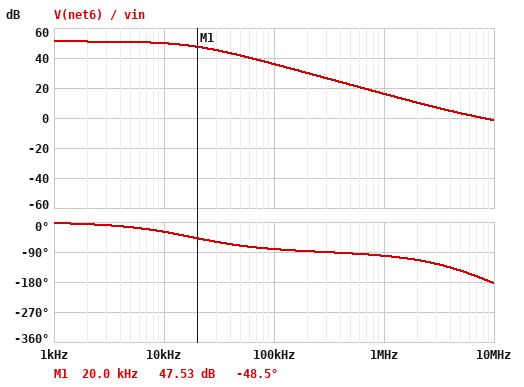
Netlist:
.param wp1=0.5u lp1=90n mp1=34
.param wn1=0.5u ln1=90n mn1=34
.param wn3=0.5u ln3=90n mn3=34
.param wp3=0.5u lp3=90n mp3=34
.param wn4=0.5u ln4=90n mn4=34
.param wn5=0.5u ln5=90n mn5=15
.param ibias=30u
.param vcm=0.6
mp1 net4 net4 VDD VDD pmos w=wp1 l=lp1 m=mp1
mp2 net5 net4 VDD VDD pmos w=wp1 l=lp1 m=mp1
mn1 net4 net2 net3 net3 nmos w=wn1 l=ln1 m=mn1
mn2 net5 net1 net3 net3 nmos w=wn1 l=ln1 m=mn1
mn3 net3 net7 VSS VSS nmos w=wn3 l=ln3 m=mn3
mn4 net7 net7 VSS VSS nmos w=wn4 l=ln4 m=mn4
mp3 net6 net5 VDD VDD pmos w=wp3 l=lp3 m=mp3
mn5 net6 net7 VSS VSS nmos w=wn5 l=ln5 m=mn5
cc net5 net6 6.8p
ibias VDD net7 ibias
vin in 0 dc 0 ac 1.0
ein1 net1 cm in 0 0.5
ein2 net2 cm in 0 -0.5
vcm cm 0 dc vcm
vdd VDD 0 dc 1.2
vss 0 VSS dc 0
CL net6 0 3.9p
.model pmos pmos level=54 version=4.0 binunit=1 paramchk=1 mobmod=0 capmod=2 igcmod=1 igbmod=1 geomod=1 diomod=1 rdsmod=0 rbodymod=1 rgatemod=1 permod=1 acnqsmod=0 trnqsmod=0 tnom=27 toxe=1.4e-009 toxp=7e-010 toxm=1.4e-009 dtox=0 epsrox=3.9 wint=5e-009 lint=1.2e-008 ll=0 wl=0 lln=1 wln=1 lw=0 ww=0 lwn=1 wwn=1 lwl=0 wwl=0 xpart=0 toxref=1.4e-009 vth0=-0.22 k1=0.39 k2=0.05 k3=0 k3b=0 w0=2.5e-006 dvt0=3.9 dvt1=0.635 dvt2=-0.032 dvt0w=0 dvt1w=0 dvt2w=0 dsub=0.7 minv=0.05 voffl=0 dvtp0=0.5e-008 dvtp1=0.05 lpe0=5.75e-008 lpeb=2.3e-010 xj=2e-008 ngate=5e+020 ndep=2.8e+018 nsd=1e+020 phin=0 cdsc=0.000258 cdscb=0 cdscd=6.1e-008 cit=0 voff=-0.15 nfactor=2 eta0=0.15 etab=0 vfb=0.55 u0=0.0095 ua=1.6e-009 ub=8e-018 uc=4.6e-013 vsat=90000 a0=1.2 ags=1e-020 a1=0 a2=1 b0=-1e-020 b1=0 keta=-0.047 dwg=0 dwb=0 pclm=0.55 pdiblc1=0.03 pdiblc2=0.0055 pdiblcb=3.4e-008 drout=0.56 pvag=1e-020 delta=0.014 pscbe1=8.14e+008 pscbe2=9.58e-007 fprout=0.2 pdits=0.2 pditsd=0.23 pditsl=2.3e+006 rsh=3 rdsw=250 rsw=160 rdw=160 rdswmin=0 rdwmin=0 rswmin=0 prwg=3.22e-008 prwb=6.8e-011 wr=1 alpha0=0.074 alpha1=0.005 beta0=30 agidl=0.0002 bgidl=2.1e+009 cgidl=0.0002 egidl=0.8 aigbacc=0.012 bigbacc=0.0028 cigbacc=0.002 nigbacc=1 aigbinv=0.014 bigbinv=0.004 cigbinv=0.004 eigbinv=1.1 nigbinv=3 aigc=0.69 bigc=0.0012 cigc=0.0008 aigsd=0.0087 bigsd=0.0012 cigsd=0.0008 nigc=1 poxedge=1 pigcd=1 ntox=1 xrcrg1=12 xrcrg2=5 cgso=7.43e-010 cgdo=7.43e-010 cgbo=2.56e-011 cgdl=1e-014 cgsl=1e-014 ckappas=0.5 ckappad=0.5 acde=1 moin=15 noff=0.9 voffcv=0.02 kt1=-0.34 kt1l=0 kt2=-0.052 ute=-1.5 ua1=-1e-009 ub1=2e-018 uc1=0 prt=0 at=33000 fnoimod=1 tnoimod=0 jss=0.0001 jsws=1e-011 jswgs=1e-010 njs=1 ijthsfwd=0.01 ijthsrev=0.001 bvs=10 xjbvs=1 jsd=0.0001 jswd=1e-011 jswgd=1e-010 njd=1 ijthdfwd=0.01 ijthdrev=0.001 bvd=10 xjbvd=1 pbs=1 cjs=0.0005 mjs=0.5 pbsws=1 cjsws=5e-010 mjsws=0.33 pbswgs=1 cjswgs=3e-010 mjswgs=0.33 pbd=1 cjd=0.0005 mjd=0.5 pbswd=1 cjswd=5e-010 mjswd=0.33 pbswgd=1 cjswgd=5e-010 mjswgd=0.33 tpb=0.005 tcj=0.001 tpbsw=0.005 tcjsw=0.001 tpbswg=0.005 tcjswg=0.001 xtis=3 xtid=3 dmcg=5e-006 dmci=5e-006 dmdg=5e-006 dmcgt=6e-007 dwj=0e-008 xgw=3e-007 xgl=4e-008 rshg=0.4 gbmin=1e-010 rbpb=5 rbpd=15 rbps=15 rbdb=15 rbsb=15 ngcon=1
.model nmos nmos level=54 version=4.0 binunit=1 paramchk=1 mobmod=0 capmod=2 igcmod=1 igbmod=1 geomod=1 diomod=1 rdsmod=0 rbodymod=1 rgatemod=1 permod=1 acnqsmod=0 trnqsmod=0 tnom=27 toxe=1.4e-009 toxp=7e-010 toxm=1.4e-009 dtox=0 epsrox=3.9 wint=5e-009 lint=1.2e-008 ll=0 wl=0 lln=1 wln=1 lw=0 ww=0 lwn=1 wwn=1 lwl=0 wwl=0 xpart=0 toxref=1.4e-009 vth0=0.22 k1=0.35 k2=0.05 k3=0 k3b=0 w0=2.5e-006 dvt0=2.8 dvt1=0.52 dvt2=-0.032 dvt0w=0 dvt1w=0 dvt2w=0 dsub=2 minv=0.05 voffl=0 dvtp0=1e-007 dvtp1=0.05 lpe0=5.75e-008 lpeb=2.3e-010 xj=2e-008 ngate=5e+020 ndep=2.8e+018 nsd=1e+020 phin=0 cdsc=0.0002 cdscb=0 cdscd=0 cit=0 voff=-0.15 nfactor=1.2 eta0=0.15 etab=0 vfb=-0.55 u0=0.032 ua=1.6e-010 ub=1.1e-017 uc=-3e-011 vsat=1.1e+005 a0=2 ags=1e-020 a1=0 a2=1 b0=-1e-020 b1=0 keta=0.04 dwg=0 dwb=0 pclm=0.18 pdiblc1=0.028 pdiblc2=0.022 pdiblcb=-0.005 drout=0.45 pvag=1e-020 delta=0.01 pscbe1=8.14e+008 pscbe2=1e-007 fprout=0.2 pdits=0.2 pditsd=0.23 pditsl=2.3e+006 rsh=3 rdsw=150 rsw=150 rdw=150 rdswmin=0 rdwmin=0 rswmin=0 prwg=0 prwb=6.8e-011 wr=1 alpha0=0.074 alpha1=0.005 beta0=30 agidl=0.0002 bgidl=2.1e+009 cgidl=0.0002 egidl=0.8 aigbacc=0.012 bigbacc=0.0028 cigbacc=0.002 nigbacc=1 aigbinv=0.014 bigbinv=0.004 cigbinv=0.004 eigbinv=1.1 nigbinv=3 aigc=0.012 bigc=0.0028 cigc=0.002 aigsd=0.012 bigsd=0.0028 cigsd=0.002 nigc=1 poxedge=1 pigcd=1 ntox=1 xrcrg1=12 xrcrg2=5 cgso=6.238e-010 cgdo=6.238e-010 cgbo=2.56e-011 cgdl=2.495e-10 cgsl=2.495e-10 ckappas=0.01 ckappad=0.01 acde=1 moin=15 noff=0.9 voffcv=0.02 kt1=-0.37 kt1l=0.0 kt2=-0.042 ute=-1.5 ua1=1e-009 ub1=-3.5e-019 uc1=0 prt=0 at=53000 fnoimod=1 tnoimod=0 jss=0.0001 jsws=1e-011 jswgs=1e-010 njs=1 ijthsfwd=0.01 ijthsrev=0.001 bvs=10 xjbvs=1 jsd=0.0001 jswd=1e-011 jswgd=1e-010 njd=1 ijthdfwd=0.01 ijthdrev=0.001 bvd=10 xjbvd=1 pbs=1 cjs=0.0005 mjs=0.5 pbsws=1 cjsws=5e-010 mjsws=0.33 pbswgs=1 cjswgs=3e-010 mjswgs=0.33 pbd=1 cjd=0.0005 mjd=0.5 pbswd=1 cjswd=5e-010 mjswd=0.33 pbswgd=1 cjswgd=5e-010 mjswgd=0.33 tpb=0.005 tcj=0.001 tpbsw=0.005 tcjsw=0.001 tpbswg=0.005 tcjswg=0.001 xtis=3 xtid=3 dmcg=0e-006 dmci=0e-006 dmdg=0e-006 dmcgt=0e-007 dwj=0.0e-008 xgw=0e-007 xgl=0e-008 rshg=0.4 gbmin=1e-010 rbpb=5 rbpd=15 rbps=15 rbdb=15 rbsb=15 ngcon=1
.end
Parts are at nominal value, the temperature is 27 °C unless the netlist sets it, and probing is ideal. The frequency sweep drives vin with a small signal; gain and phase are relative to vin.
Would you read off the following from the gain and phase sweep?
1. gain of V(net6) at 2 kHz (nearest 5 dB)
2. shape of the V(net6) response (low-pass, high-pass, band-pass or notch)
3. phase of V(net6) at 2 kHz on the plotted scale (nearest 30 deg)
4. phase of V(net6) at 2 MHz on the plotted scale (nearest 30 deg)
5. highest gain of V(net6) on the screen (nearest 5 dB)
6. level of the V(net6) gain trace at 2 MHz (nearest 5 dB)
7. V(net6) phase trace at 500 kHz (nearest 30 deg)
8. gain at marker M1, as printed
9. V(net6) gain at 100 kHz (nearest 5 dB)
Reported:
50 dB
low-pass
0 deg
-120 deg
50 dB
10 dB
-90 deg
47.53 dB
35 dB
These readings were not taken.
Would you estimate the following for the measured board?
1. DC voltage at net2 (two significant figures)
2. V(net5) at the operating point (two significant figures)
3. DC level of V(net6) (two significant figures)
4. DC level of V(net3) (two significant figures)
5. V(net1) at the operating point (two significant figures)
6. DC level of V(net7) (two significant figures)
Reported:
600 mV
880 mV
650 mV
320 mV
600 mV
320 mV
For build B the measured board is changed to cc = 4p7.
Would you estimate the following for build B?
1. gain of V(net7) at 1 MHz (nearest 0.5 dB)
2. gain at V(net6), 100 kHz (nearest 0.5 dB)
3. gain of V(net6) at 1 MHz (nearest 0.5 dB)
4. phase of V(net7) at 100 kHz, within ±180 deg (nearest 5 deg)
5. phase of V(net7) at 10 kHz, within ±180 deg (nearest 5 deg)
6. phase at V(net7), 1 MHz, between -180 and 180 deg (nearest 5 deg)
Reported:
-48.5 dB
39.0 dB
19.0 dB
-75 deg
-20 deg
-90 deg
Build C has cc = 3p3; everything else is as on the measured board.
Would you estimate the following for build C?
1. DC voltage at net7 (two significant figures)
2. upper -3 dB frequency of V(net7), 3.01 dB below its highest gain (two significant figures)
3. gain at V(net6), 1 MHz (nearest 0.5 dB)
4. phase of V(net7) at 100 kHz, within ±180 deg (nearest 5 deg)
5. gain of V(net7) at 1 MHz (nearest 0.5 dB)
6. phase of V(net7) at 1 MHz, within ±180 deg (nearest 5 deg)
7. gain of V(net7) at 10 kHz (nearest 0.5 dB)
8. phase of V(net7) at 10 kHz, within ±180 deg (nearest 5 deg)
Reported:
320 mV
36 kHz
22.0 dB
-70 deg
-45.5 dB
-90 deg
-17.0 dB
-15 deg
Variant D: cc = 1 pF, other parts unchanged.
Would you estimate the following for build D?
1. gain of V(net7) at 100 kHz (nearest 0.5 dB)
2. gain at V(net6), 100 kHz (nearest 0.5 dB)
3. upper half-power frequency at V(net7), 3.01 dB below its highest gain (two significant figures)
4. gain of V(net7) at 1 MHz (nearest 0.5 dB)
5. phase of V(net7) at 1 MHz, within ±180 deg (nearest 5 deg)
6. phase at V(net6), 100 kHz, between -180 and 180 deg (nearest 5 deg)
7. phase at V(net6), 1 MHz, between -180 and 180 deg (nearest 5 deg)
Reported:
-19.5 dB
48.0 dB
100 kHz
-36.5 dB
-80 deg
-45 deg
-90 deg
